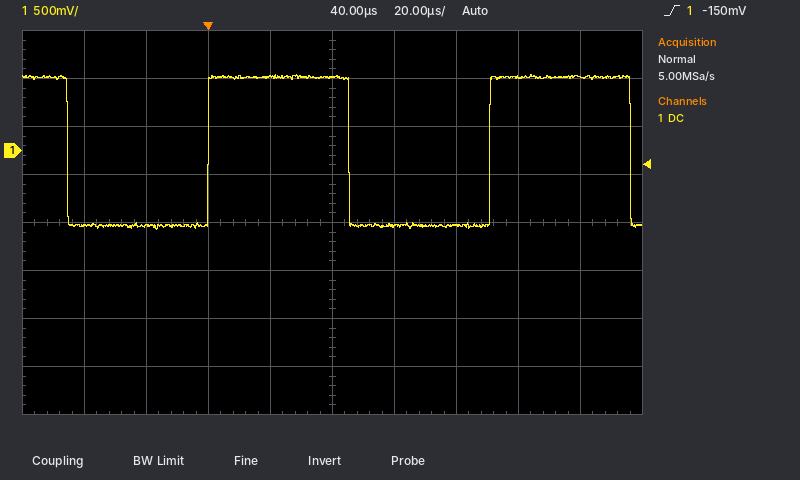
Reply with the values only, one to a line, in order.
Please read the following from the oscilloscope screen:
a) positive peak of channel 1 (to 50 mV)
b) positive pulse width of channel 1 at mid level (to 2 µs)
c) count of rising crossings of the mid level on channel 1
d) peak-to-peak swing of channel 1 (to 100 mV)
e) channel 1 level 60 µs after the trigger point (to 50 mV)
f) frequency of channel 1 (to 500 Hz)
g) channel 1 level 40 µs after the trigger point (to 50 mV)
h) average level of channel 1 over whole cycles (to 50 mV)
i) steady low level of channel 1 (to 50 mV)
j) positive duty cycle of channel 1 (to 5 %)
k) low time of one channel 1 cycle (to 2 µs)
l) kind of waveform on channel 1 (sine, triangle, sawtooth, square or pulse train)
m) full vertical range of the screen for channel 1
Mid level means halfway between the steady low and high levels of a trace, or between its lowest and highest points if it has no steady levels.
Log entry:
800 mV
46 µs
2
1.60 V
-800 mV
11.0 kHz
750 mV
0 mV
-800 mV
50 %
46 µs
square
4 V
